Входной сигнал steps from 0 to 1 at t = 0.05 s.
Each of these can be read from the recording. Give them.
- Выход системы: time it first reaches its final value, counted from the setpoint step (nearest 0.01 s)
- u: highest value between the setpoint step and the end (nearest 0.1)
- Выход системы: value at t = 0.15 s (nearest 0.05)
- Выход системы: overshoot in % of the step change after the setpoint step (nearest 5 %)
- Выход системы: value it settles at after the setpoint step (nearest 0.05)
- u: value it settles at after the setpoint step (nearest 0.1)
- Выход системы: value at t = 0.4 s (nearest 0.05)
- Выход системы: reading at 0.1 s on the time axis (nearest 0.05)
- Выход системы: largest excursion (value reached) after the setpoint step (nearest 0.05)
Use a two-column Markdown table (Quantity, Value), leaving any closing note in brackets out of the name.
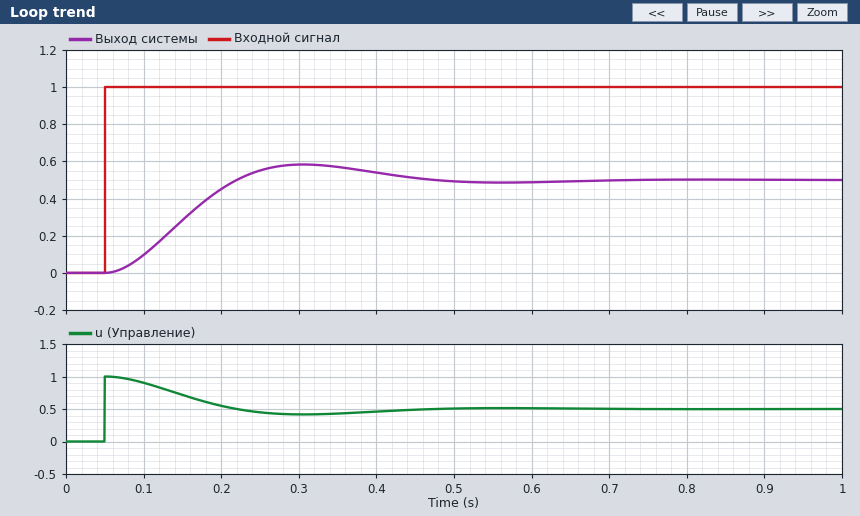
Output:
| Quantity | Value |
|---|---|
| Выход системы: time it first reaches its final value, counted from the setpoint step | 0.17 s |
| u: highest value between the setpoint step and the end | 1.0 |
| Выход системы: value at t = 0.15 s | 0.30 |
| Выход системы: overshoot in % of the step change after the setpoint step | 15 % |
| Выход системы: value it settles at after the setpoint step | 0.50 |
| u: value it settles at after the setpoint step | 0.5 |
| Выход системы: value at t = 0.4 s | 0.55 |
| Выход системы: reading at 0.1 s on the time axis | 0.10 |
| Выход системы: largest excursion (value reached) after the setpoint step | 0.60 |
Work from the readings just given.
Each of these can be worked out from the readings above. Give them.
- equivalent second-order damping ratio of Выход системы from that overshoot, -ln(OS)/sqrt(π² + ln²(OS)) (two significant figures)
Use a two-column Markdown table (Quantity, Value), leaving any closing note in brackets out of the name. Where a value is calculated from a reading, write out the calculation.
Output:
| Quantity | Value |
|---|---|
| equivalent second-order damping ratio of Выход системы from that overshoot, -ln(OS)/sqrt(π² + ln²(OS)) | ln(0.15) = -1.897; 1.897 / sqrt(9.870 + 3.599) = 0.52 |
